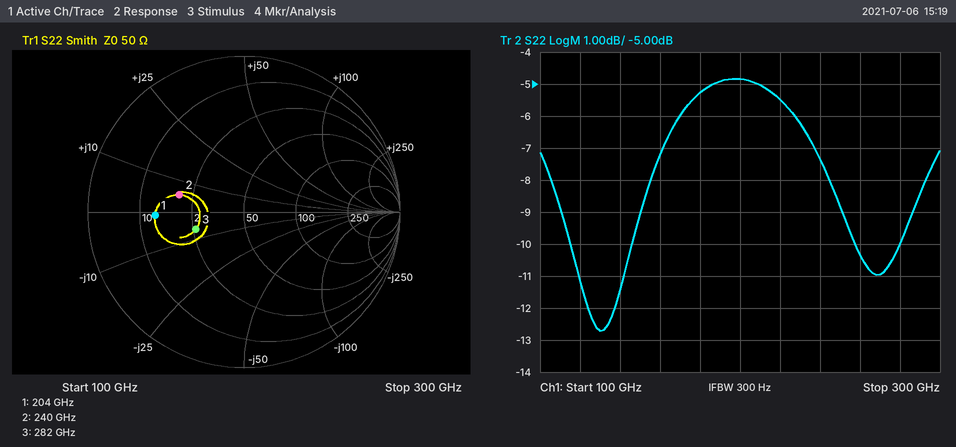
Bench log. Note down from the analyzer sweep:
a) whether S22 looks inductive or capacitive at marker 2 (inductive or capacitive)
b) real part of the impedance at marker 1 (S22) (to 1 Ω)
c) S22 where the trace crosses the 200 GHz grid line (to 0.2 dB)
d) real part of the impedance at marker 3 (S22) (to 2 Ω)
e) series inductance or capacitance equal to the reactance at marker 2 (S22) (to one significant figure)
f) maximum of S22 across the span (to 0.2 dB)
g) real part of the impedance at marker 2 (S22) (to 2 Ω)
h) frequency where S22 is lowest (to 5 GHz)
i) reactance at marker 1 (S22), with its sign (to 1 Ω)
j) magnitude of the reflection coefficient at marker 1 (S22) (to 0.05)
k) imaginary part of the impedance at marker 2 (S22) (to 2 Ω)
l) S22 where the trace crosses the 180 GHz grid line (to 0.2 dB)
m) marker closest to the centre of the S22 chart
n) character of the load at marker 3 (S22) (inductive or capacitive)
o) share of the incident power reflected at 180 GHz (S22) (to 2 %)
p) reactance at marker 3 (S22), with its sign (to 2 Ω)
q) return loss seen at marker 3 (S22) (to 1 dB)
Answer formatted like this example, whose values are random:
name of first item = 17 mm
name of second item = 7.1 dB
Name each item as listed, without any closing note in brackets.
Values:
whether S22 looks inductive or capacitive at marker 2 = inductive
real part of the impedance at marker 1 (S22) = 14 Ω
S22 where the trace crosses the 200 GHz grid line = -4.8 dB
real part of the impedance at marker 3 (S22) = 26 Ω
series inductance or capacitance equal to the reactance at marker 2 (S22) = 4 pH
maximum of S22 across the span = -4.8 dB
real part of the impedance at marker 2 (S22) = 20 Ω
frequency where S22 is lowest = 130 GHz
reactance at marker 1 (S22), with its sign = -1 Ω
magnitude of the reflection coefficient at marker 1 (S22) = 0.55
imaginary part of the impedance at marker 2 (S22) = +6 Ω
S22 where the trace crosses the 180 GHz grid line = -5.2 dB
marker closest to the centre of the S22 chart = marker 3
character of the load at marker 3 (S22) = capacitive
share of the incident power reflected at 180 GHz (S22) = 30 %
reactance at marker 3 (S22), with its sign = -6 Ω
return loss seen at marker 3 (S22) = 10 dB
